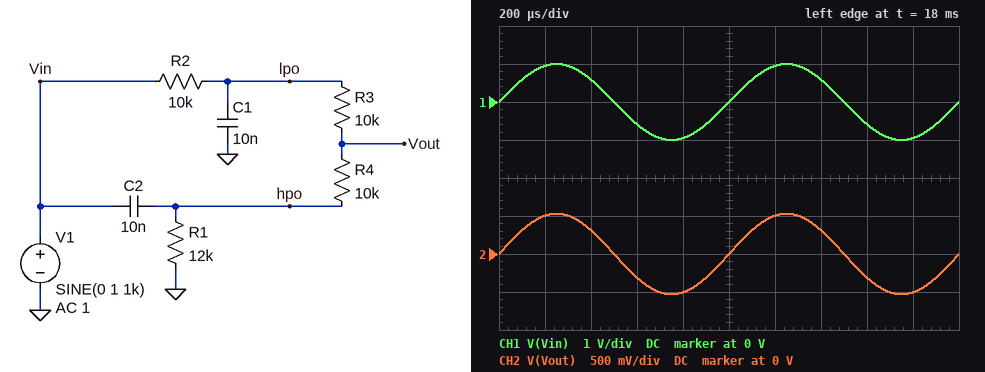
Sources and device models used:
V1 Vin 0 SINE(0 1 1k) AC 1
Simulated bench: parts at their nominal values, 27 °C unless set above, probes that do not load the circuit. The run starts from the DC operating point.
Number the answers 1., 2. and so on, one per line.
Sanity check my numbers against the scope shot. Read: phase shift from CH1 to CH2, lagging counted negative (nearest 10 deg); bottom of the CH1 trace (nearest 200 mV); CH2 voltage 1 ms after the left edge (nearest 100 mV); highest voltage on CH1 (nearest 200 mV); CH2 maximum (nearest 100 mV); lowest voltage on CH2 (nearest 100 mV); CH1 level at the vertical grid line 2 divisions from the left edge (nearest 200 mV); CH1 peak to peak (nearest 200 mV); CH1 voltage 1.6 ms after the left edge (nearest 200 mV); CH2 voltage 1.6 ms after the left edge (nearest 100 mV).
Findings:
1. 0 deg
2. -1.0 V
3. 0 V
4. 1.0 V
5. 500 mV
6. -500 mV
7. 600 mV
8. 2.0 V
9. -600 mV
10. -300 mV
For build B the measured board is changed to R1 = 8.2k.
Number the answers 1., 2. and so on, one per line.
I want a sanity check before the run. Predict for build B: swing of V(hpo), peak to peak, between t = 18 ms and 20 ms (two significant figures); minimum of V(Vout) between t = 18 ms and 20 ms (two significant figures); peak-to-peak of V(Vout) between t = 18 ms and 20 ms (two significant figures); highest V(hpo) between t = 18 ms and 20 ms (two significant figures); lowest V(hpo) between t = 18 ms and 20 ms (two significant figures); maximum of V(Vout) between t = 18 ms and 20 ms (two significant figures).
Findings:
1. 680 mV
2. -470 mV
3. 940 mV
4. 340 mV
5. -340 mV
6. 470 mV
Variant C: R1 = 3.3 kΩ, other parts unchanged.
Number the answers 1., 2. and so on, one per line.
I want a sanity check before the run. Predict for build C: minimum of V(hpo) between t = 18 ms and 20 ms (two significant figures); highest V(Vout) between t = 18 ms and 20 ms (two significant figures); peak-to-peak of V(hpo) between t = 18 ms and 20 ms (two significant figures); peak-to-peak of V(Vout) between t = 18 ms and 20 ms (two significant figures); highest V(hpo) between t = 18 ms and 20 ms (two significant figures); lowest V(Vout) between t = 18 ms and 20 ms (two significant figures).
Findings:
1. -170 mV
2. 360 mV
3. 340 mV
4. 730 mV
5. 170 mV
6. -360 mV
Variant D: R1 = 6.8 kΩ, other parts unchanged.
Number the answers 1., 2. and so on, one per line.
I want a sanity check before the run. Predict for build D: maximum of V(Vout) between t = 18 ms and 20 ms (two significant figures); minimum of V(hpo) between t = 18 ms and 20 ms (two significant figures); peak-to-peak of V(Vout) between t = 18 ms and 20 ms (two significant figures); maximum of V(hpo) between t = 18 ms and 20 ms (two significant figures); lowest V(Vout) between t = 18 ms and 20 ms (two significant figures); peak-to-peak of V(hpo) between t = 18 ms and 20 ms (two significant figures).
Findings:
1. 440 mV
2. -300 mV
3. 880 mV
4. 300 mV
5. -440 mV
6. 600 mV
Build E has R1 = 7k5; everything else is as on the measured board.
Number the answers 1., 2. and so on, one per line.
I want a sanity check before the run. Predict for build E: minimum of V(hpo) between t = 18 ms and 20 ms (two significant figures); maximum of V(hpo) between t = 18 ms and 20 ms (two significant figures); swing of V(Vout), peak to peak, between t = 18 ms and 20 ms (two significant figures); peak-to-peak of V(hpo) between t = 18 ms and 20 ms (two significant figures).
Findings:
1. -320 mV
2. 320 mV
3. 910 mV
4. 640 mV
